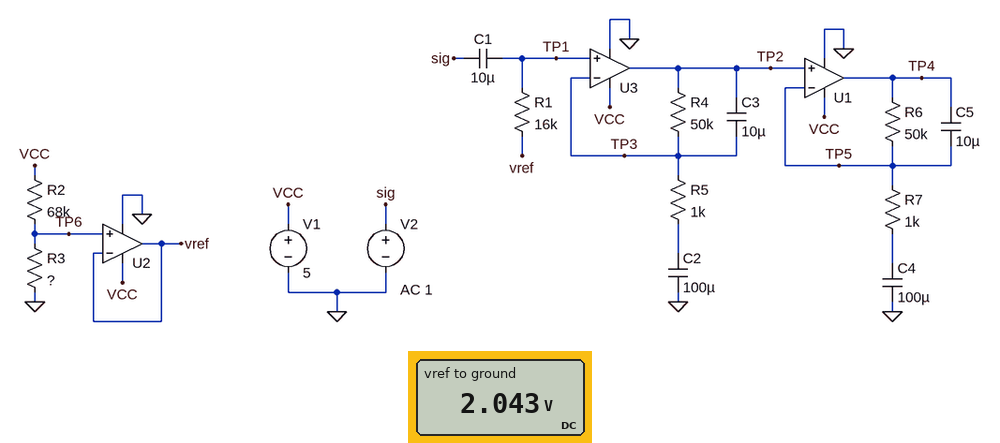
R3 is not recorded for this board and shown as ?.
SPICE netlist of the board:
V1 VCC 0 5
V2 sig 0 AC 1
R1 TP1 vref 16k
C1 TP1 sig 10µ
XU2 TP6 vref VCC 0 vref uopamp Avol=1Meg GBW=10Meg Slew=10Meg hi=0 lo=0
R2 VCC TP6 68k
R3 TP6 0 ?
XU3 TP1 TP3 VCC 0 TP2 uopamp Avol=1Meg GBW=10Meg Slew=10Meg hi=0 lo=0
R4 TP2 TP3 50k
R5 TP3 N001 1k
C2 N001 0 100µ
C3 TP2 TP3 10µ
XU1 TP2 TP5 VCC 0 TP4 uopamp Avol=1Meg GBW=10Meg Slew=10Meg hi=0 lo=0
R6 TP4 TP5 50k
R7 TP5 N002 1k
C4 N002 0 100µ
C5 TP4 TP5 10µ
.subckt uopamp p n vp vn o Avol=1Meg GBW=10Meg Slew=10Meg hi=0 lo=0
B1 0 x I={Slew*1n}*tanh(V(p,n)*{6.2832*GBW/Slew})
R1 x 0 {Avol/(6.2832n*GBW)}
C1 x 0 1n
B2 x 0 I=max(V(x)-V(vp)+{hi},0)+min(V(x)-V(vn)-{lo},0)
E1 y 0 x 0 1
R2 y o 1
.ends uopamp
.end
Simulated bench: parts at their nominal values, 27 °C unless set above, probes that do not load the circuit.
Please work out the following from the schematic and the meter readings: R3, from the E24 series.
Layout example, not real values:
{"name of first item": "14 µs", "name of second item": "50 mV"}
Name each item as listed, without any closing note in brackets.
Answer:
{"R3, from the E24 series": "47 kΩ"}
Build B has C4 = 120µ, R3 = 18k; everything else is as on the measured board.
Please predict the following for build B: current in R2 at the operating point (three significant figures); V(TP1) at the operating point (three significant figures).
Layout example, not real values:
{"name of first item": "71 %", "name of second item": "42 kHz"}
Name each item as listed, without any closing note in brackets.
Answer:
{"current in R2 at the operating point": "58.1 µA", "V(TP1) at the operating point": "1.05 V"}
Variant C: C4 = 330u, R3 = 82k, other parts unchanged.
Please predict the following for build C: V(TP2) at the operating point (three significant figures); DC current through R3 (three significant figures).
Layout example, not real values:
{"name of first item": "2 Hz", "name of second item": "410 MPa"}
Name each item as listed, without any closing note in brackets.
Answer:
{"V(TP2) at the operating point": "2.73 V", "DC current through R3": "33.3 µA"}
